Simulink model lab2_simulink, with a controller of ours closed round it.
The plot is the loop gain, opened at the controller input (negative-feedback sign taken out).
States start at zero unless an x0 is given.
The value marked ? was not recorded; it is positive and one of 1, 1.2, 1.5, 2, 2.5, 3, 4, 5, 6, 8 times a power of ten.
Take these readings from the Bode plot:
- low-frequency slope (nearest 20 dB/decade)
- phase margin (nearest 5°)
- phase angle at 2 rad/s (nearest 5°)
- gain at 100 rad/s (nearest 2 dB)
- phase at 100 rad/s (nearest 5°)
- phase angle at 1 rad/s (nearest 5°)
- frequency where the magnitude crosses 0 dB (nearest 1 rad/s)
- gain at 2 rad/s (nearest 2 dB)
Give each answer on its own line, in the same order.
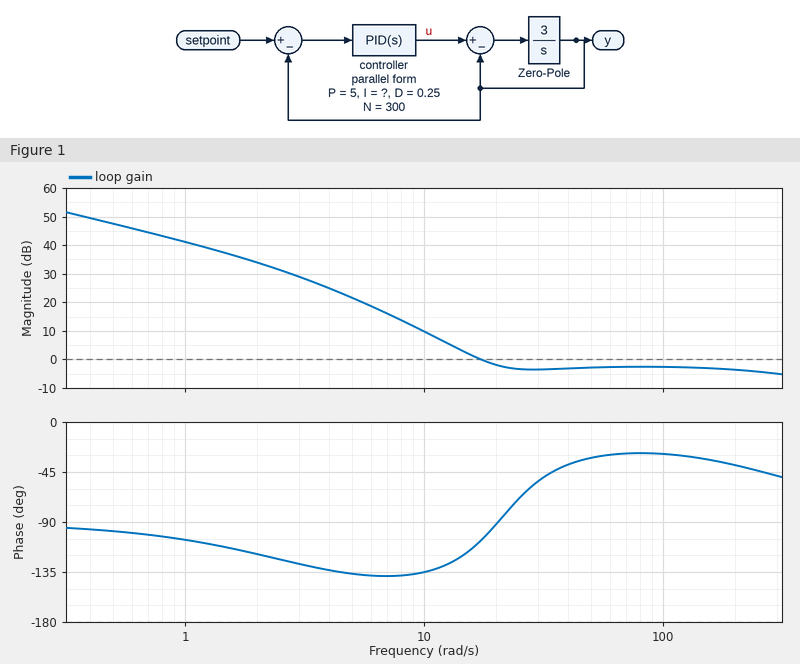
-20 dB/decade
75°
-120°
-2 dB
-30°
-105°
17 rad/s
34 dB
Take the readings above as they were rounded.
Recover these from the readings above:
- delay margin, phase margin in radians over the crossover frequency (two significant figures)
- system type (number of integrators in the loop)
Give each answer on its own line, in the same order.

0.077 s
1
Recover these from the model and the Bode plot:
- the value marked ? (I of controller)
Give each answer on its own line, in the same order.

120
